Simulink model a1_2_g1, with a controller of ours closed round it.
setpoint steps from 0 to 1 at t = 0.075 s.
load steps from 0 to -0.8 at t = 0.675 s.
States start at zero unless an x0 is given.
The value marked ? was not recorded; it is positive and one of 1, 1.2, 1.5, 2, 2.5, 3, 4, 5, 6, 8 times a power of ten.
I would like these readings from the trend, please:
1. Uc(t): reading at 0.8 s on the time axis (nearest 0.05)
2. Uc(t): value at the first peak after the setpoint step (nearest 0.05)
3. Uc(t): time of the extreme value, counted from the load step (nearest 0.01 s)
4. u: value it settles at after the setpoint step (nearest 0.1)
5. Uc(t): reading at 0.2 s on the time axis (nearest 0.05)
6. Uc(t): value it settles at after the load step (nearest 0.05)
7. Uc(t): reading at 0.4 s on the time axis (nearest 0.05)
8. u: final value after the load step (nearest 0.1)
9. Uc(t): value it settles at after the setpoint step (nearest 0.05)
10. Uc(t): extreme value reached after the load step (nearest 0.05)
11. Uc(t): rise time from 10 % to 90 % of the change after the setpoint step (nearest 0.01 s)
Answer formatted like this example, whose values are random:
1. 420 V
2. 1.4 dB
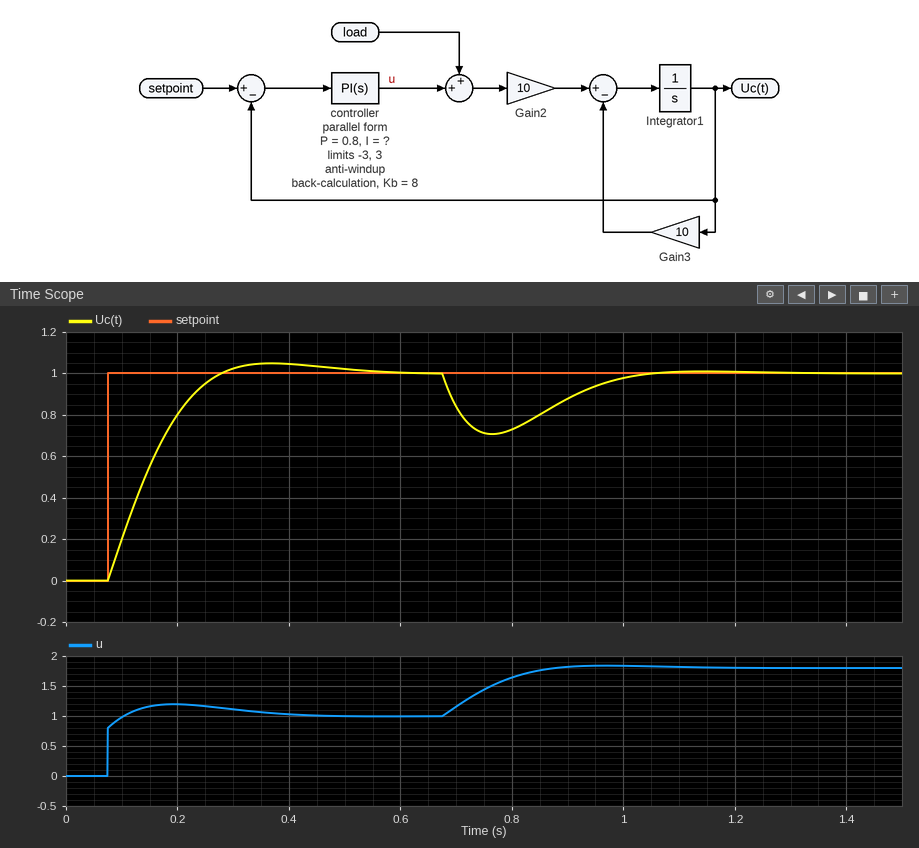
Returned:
1. 0.75
2. 1.05
3. 0.09 s
4. 1.0
5. 0.80
6. 1.00
7. 1.05
8. 1.8
9. 1.00
10. 0.70
11. 0.14 s
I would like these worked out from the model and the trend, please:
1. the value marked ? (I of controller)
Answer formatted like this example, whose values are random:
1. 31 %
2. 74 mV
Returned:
1. 15
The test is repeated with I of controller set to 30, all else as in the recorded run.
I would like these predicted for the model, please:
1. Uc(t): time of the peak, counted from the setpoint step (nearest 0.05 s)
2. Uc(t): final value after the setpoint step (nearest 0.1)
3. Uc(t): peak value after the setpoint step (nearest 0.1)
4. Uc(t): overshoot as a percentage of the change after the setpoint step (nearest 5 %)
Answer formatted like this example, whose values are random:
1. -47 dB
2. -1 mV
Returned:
1. 0.20 s
2. 1.0
3. 1.2
4. 15 %
